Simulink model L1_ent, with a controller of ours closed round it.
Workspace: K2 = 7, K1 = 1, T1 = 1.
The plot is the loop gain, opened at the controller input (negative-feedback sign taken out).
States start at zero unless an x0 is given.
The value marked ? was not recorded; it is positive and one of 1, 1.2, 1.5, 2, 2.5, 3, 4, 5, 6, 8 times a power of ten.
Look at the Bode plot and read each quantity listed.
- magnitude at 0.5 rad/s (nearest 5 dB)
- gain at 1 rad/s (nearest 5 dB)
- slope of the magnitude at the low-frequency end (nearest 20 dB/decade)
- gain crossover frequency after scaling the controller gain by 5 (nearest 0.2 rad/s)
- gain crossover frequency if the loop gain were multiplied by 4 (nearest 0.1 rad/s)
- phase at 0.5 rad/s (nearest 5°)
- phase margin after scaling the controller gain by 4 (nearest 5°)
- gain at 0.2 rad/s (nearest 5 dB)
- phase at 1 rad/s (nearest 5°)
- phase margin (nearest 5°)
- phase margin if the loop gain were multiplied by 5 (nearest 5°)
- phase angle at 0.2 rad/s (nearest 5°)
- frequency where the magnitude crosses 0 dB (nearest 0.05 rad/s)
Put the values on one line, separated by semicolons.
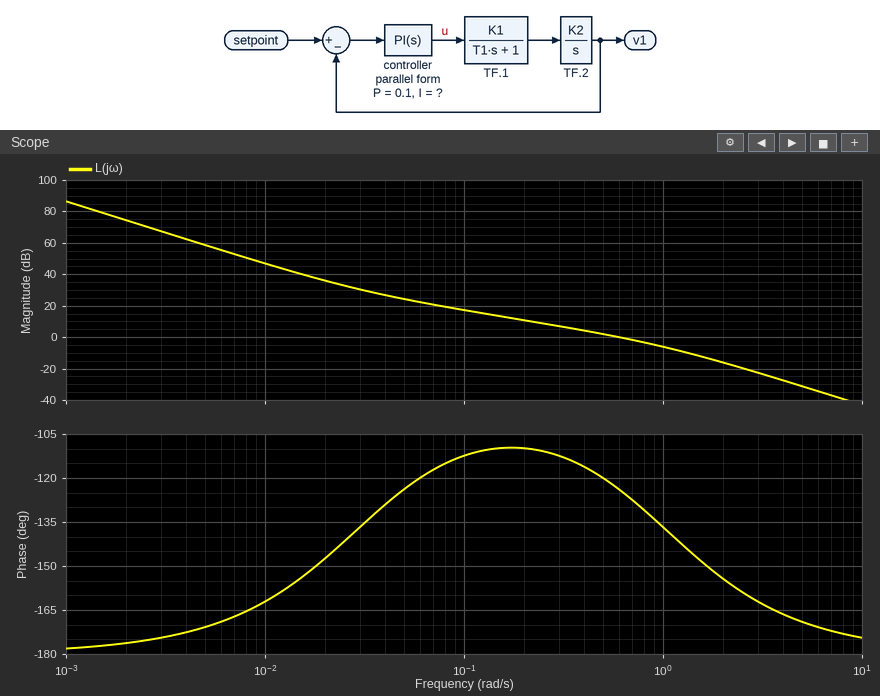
0 dB; -5 dB; -40 dB/decade; 1.8 rad/s; 1.5 rad/s; -120°; 30°; 10 dB; -135°; 55°; 30°; -110°; 0.60 rad/s
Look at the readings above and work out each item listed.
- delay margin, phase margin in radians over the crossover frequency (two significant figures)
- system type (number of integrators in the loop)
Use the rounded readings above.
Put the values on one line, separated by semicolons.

1.6 s; 2
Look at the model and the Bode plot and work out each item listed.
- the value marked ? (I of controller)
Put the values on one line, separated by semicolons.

0.003
